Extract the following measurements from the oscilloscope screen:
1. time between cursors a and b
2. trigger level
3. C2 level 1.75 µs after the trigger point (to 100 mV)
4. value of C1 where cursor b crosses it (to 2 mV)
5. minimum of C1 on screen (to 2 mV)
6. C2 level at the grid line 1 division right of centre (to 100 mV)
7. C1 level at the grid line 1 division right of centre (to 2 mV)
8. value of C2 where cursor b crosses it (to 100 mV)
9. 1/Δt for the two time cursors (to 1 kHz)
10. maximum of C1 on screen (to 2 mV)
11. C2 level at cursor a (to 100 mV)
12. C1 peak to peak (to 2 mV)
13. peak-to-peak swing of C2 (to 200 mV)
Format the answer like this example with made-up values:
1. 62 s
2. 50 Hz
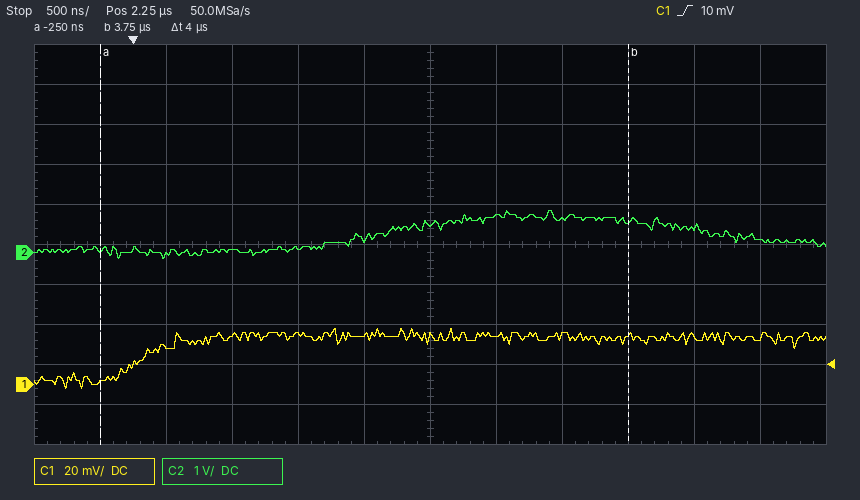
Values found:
1. 4 µs
2. 10 mV
3. 300 mV
4. 24 mV
5. -2 mV
6. 900 mV
7. 24 mV
8. 800 mV
9. 250 kHz
10. 28 mV
11. 100 mV
12. 30 mV
13. 1.2 V
